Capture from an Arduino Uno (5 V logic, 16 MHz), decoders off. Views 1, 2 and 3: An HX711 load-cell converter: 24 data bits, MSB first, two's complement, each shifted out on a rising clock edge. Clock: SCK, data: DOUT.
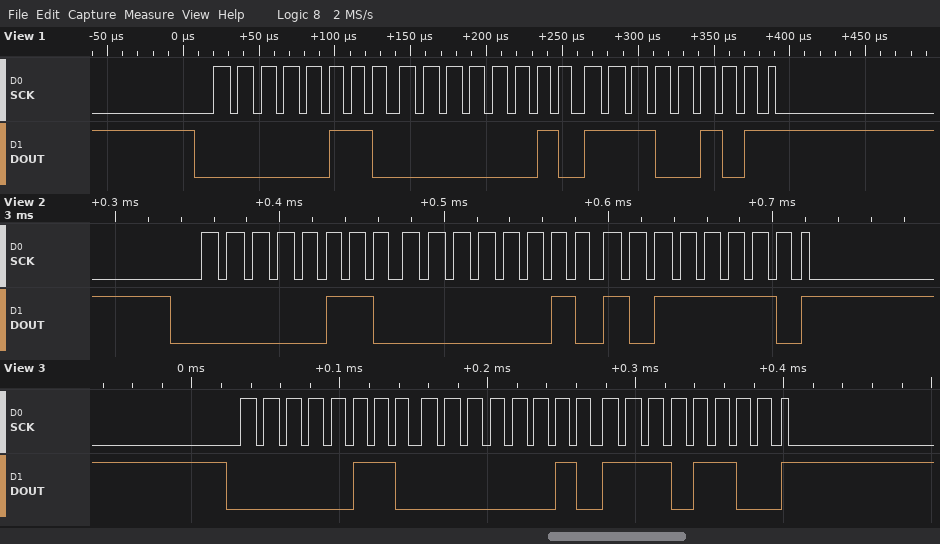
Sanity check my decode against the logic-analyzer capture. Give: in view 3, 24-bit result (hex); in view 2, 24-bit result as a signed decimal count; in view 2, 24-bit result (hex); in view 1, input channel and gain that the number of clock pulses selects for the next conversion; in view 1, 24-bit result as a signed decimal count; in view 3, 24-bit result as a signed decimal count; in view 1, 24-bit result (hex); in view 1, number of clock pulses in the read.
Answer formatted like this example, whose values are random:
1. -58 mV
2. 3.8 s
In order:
1. 0x0602EC
2. 393918
3. 0x0602BE
4. channel A, gain 128
5. 393957
6. 393964
7. 0x0602E5
8. 25
